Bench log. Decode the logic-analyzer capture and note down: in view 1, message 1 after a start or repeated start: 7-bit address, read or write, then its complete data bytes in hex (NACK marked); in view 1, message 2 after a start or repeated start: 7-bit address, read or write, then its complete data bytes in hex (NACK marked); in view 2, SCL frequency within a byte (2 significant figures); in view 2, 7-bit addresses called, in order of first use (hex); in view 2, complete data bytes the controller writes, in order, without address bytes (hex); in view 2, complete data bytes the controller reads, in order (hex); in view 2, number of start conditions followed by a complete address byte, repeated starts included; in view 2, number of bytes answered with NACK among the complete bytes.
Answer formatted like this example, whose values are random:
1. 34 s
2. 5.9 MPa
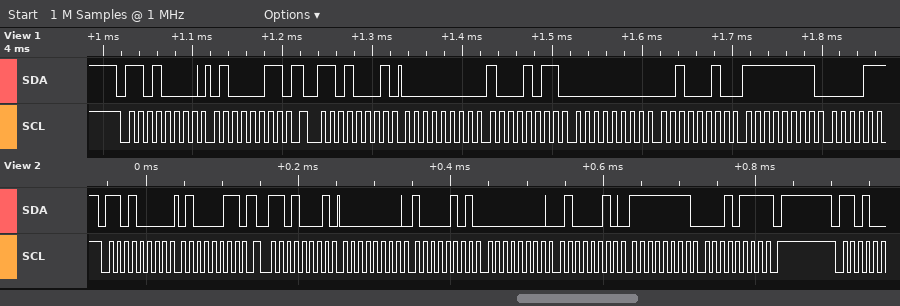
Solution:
1. 0x68 write: 43
2. 0x68 read: 00 8B 00 22 FF
3. 100 kHz
4. 0x68
5. 43
6. 00 85 00 42 FF 17
7. 2
8. 1
